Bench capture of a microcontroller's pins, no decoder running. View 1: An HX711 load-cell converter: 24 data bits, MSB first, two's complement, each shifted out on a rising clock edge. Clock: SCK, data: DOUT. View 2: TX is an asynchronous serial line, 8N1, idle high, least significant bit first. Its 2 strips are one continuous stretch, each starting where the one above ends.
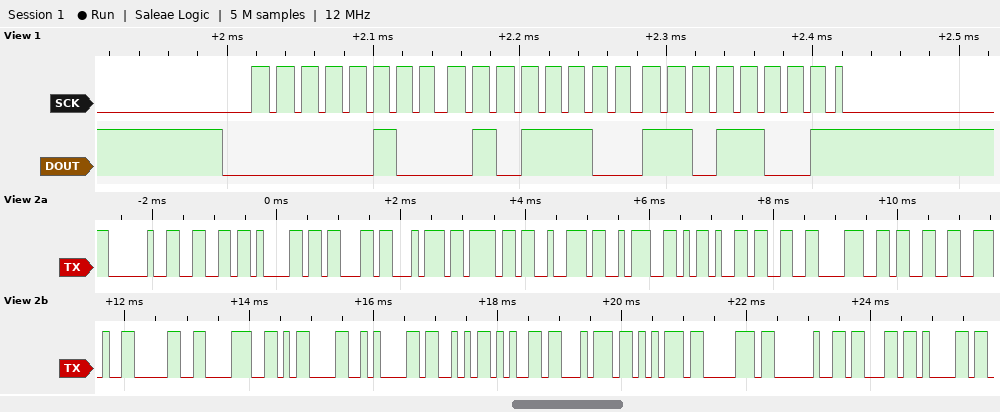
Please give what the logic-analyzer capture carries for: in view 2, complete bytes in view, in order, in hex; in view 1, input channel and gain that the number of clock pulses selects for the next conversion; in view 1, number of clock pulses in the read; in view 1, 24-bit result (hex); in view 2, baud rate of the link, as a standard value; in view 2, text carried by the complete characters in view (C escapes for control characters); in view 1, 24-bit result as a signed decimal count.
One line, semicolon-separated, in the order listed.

20 66 61 63 74 6F 72 3A 2D 33 38 33 2E 30 38 0D 0A 53 65 74 75 70 20 63 61; channel A, gain 128; 25; 0x045CD9; 9600 baud; " factor:-383.08\r\nSetup ca"; 285913
